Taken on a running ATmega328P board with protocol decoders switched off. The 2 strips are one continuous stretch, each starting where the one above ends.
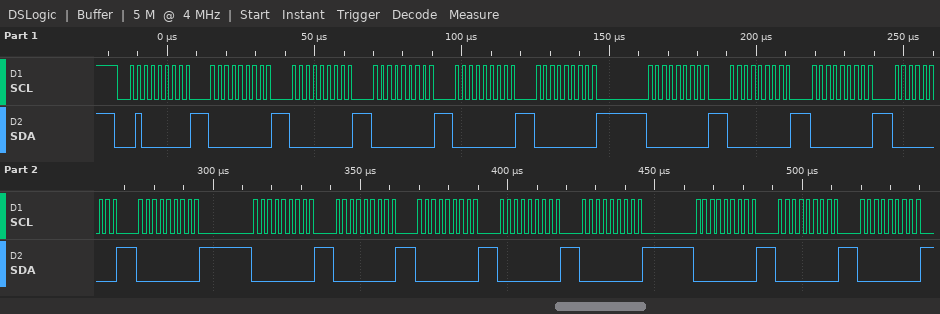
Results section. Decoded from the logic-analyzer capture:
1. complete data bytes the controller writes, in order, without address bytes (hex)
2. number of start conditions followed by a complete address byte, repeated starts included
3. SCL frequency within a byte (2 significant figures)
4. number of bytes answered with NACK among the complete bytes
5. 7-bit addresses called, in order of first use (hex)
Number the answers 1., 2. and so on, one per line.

1. 00 00 00 00 00 00 00 00 00 00 00 00 00 00 00 00 00 00
2. 1
3. 420 kHz
4. 0
5. 0x20
